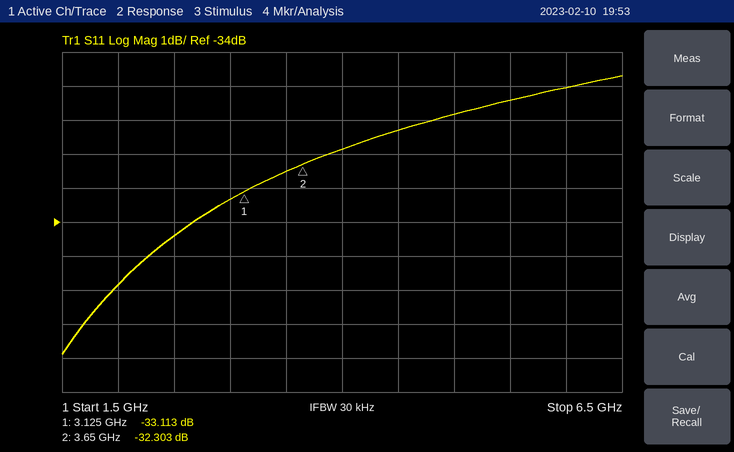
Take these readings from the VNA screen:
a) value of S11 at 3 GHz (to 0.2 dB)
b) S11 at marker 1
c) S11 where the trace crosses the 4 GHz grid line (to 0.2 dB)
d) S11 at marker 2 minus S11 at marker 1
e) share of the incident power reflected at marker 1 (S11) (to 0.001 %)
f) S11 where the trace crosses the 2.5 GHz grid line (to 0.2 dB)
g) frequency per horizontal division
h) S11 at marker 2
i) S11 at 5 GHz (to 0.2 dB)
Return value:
-33.4 dB
-33.113 dB
-31.8 dB
0.810 dB
0.049 %
-34.4 dB
500 MHz
-32.303 dB
-30.8 dB
